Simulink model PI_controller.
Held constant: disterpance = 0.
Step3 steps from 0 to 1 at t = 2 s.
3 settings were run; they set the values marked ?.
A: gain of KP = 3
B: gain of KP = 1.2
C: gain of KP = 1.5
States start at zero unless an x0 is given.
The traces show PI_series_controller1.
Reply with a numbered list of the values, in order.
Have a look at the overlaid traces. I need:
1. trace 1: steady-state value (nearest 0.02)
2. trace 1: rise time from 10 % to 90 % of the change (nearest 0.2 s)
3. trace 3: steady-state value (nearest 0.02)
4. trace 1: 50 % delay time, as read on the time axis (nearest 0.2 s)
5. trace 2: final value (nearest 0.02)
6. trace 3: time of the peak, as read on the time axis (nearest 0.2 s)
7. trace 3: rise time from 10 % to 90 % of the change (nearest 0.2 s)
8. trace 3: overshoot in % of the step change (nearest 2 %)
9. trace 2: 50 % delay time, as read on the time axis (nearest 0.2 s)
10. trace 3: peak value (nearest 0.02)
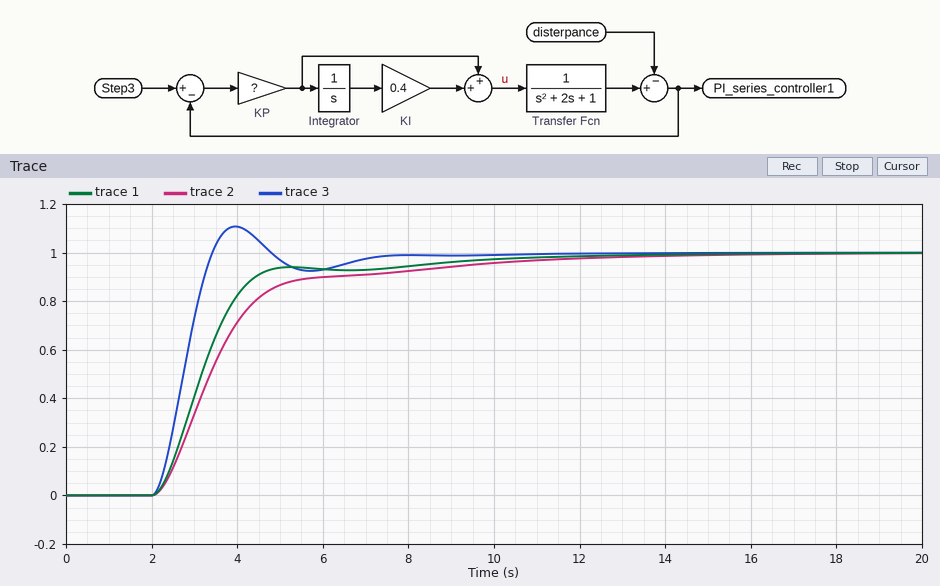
1. 1.00
2. 2.0 s
3. 1.00
4. 3.2 s
5. 1.00
6. 4.0 s
7. 1.0 s
8. 10 %
9. 3.4 s
10. 1.10
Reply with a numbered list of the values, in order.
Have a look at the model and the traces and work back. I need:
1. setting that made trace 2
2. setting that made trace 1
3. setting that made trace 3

1. B
2. C
3. A
